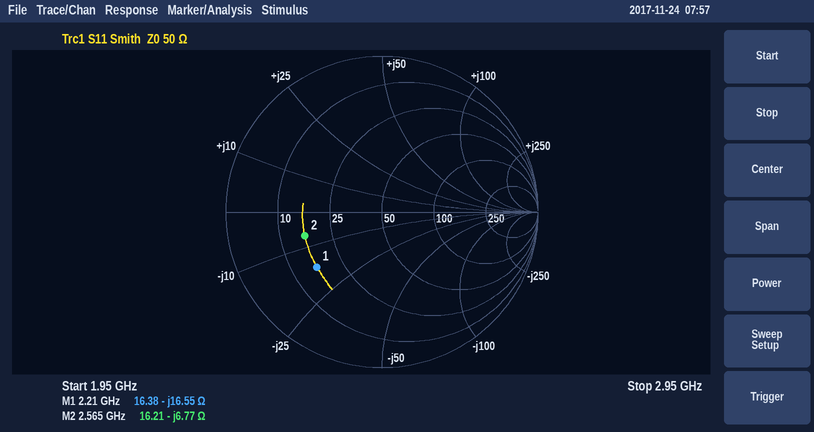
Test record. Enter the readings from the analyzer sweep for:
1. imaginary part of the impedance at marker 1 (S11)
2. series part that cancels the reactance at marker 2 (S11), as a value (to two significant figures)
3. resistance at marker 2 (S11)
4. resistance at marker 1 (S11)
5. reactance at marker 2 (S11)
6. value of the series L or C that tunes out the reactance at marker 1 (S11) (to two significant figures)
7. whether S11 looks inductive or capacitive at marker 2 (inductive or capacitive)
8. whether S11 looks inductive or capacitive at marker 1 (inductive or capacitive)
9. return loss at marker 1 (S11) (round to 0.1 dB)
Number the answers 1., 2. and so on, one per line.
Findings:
1. -16.55 Ω
2. 420 pH
3. 16.21 Ω
4. 16.38 Ω
5. -6.77 Ω
6. 1.2 nH
7. capacitive
8. capacitive
9. 5.2 dB
